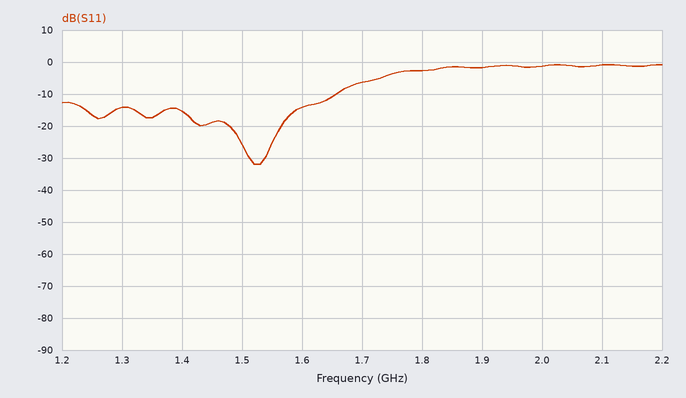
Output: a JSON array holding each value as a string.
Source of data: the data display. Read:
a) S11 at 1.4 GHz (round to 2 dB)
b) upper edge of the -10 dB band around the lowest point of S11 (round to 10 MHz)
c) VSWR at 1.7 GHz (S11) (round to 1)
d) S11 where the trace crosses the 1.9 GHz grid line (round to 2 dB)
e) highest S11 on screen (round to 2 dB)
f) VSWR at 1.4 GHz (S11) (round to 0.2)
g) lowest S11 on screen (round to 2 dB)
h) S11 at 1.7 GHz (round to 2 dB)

["-16 dB", "1.66 GHz", "3", "-2 dB", "0 dB", "1.4", "-32 dB", "-6 dB"]
